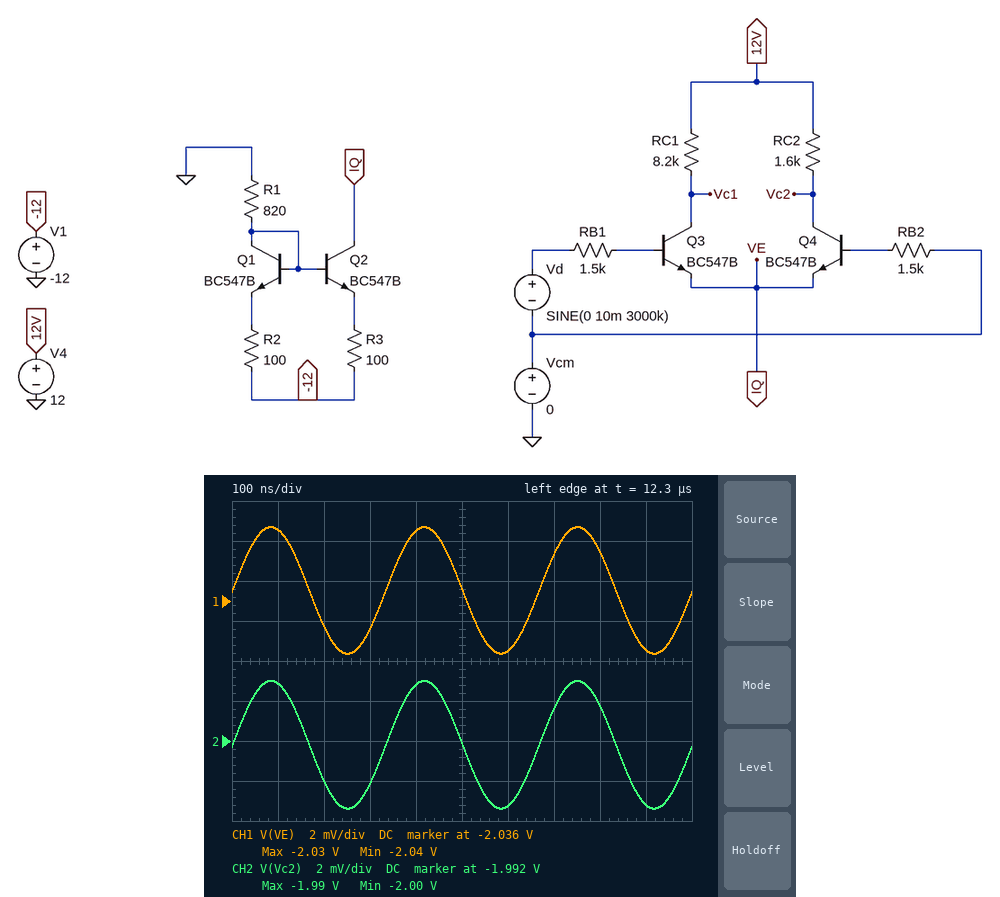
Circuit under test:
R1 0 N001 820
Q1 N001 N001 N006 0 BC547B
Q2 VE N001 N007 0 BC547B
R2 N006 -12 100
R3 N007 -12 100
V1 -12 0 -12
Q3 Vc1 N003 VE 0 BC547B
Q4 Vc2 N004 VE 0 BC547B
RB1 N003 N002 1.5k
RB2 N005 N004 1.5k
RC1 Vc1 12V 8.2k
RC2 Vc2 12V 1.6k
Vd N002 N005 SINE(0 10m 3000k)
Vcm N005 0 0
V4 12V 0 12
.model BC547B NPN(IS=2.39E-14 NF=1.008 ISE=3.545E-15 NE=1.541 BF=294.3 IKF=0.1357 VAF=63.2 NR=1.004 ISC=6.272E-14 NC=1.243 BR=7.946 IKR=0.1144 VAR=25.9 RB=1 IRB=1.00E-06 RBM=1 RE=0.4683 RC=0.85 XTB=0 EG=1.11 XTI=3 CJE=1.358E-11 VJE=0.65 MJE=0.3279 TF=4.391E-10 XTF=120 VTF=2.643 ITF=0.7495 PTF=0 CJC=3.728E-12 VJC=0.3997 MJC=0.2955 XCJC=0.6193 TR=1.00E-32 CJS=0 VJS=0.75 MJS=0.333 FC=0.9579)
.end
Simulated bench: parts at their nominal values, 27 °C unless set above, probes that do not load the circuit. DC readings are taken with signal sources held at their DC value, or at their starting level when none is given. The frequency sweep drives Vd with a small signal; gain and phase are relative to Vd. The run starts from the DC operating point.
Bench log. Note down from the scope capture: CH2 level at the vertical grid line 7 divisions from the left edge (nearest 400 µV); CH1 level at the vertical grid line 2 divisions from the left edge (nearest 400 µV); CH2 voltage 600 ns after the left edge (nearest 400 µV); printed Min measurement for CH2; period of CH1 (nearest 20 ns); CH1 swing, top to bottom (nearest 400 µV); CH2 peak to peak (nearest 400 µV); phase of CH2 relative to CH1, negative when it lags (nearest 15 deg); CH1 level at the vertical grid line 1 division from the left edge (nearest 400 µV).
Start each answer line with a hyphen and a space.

- -1.9904 V
- -2.0372 V
- -1.9952 V
- -2.00 V
- 340 ns
- 6.4 mV
- 6.4 mV
- 0 deg
- -2.0324 V
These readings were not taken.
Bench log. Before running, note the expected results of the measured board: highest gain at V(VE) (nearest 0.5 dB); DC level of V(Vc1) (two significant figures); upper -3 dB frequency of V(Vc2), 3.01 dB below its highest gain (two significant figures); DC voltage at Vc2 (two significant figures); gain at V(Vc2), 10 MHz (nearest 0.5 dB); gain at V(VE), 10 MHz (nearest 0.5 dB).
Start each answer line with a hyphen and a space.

- -10.0 dB
- -2.0 V
- 96 MHz
- -2.0 V
- -10.0 dB
- -10.0 dB
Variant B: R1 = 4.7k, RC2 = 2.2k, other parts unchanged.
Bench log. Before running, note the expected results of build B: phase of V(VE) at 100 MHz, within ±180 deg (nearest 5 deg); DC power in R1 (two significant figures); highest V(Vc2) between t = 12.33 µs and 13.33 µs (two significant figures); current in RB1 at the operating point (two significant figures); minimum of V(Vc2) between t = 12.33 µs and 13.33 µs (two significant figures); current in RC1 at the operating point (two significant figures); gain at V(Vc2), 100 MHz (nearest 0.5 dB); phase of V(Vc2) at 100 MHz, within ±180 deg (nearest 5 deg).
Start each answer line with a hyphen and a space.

- -30 deg
- 26 mW
- 9.3 V
- 3.8 µA
- 9.2 V
- 1.1 mA
- -16.0 dB
- -50 deg
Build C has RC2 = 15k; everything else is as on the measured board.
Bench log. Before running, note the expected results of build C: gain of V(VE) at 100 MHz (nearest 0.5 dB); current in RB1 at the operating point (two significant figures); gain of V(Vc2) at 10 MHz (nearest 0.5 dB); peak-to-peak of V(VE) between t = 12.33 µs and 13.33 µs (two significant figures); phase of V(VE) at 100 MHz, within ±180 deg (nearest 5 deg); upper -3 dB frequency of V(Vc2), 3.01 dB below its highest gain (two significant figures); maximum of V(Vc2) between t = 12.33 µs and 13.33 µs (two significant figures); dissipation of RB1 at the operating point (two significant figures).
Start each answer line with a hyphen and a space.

- -13.0 dB
- 4.3 mA
- -7.5 dB
- 8.7 mV
- -40 deg
- 53 MHz
- -7.2 V
- 28 mW
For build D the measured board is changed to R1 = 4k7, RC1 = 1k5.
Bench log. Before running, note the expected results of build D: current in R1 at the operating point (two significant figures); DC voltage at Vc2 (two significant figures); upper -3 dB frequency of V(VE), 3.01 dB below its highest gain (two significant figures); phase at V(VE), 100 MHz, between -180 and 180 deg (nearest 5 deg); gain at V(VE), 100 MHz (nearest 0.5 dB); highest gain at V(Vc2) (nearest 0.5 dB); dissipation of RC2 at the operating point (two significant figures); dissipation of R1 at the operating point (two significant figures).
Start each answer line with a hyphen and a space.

- 2.4 mA
- 10 V
- 49 MHz
- -45 deg
- -13.0 dB
- 29.0 dB
- 2.3 mW
- 26 mW
